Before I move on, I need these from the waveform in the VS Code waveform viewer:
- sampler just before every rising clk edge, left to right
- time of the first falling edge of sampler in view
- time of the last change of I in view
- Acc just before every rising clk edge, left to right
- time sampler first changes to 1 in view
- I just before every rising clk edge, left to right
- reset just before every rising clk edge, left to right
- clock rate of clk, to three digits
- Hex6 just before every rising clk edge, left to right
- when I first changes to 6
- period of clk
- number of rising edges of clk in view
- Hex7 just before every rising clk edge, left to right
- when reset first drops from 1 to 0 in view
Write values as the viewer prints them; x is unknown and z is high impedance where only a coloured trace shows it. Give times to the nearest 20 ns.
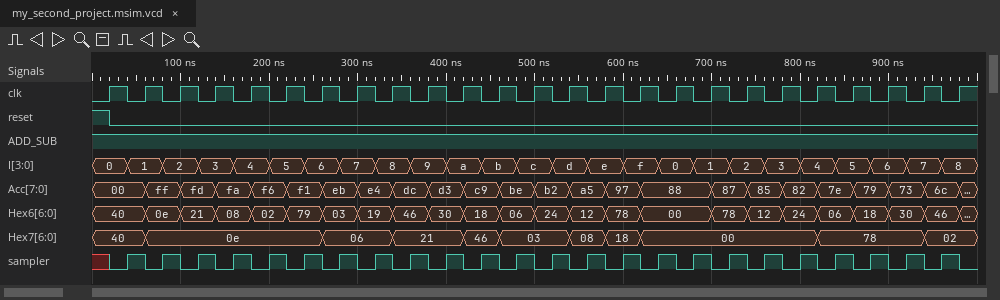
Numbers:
x 1 1 1 1 1 1 1 1 1 1 1 1 1 1 1 1 1 1 1 1 1 1 1 1
60 ns
960 ns
00, 00, ff, fd, fa, f6, f1, eb, e4, dc, d3, c9, be, b2, a5, 97, 88, 88, 87, 85, 82, 7e, 79, 73, 6c
40 ns
0, 1, 2, 3, 4, 5, 6, 7, 8, 9, a, b, c, d, e, f, 0, 1, 2, 3, 4, 5, 6, 7, 8
1 0 0 0 0 0 0 0 0 0 0 0 0 0 0 0 0 0 0 0 0 0 0 0 0
25.0 MHz
40, 40, 0e, 21, 08, 02, 79, 03, 19, 46, 30, 18, 06, 24, 12, 78, 00, 00, 78, 12, 24, 06, 18, 30, 46
240 ns
40 ns
25
40, 40, 0e, 0e, 0e, 0e, 0e, 06, 06, 21, 21, 46, 03, 03, 08, 18, 00, 00, 00, 00, 00, 78, 78, 78, 02
20 ns
